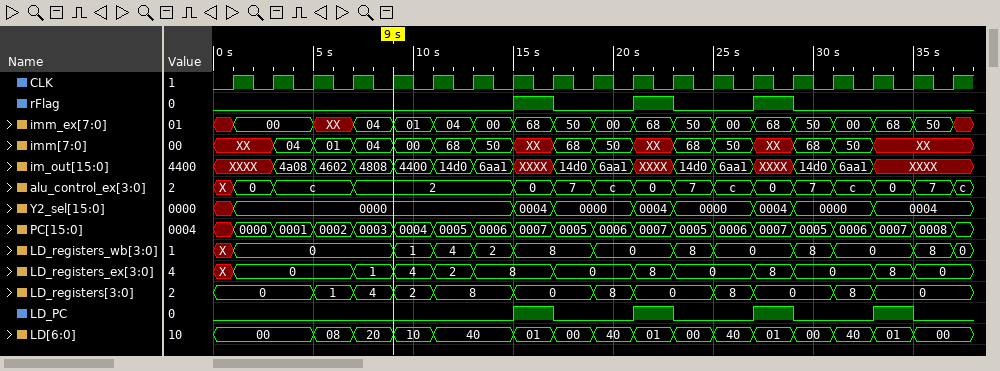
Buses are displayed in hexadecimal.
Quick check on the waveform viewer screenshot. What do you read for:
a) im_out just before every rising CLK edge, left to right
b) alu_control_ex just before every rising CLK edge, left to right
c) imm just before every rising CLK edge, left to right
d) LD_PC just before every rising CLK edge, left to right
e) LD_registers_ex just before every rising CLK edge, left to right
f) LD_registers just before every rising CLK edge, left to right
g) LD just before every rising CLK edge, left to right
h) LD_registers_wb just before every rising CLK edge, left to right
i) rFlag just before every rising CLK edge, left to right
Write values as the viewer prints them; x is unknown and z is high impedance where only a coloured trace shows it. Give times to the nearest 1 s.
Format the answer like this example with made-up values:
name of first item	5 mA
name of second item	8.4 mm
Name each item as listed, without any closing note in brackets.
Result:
im_out just before every rising CLK edge, left to right	XXXX, XXXX, 4a08, 4602, 4808, 4400, 14d0, 6aa1, XXXX, 14d0, 6aa1, XXXX, 14d0, 6aa1, XXXX, 14d0, 6aa1, XXXX, XXXX
alu_control_ex just before every rising CLK edge, left to right	X, 0, c, c, 2, 2, 2, 2, 0, 7, c, 0, 7, c, 0, 7, c, 0, 7
imm just before every rising CLK edge, left to right	XX, XX, 04, 01, 04, 00, 68, 50, XX, 68, 50, XX, 68, 50, XX, 68, 50, XX, XX
LD_PC just before every rising CLK edge, left to right	0 0 0 0 0 0 0 0 1 0 0 1 0 0 1 0 0 1 0
LD_registers_ex just before every rising CLK edge, left to right	X, 0, 0, 0, 1, 4, 2, 8, 8, 0, 0, 8, 0, 0, 8, 0, 0, 8, 0
LD_registers just before every rising CLK edge, left to right	0, 0, 0, 1, 4, 2, 8, 8, 0, 0, 8, 0, 0, 8, 0, 0, 8, 0, 0
LD just before every rising CLK edge, left to right	00, 00, 00, 08, 20, 10, 40, 40, 01, 00, 40, 01, 00, 40, 01, 00, 40, 01, 00
LD_registers_wb just before every rising CLK edge, left to right	X, 0, 0, 0, 0, 1, 4, 2, 8, 8, 0, 0, 8, 0, 0, 8, 0, 0, 8
rFlag just before every rising CLK edge, left to right	0 0 0 0 0 0 0 0 1 0 0 1 0 0 1 0 0 0 0
